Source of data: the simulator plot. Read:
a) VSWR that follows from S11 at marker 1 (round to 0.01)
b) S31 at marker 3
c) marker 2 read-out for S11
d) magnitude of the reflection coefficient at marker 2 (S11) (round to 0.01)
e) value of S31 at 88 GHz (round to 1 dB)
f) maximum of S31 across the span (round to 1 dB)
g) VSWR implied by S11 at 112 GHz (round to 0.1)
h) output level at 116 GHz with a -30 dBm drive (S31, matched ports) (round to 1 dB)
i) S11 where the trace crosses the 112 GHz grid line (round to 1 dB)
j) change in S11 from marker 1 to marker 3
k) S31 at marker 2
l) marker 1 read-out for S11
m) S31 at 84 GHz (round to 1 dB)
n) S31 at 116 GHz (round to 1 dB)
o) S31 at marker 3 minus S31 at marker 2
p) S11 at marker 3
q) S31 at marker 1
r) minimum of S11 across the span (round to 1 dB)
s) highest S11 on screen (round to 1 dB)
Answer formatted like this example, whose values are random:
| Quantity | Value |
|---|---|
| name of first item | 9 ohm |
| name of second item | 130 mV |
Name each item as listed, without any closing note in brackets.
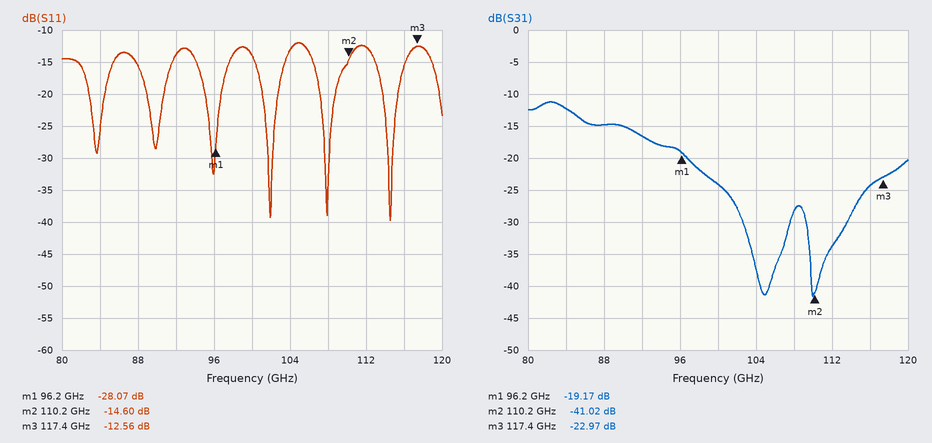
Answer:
| Quantity | Value |
|---|---|
| VSWR that follows from S11 at marker 1 | 1.08 |
| S31 at marker 3 | -22.97 dB |
| marker 2 read-out for S11 | -14.60 dB |
| magnitude of the reflection coefficient at marker 2 (S11) | 0.19 |
| value of S31 at 88 GHz | -15 dB |
| maximum of S31 across the span | -11 dB |
| VSWR implied by S11 at 112 GHz | 1.6 |
| output level at 116 GHz with a -30 dBm drive (S31, matched ports) | -54 dBm |
| S11 where the trace crosses the 112 GHz grid line | -13 dB |
| change in S11 from marker 1 to marker 3 | 15.51 dB |
| S31 at marker 2 | -41.02 dB |
| marker 1 read-out for S11 | -28.07 dB |
| S31 at 84 GHz | -12 dB |
| S31 at 116 GHz | -24 dB |
| S31 at marker 3 minus S31 at marker 2 | 18.05 dB |
| S11 at marker 3 | -12.56 dB |
| S31 at marker 1 | -19.17 dB |
| minimum of S11 across the span | -40 dB |
| highest S11 on screen | -12 dB |
